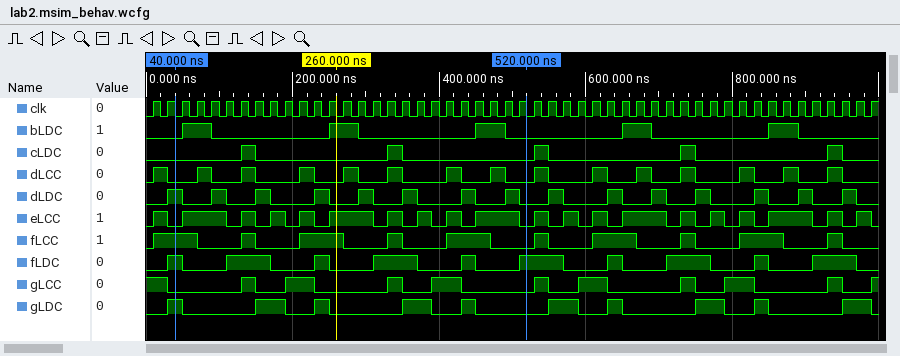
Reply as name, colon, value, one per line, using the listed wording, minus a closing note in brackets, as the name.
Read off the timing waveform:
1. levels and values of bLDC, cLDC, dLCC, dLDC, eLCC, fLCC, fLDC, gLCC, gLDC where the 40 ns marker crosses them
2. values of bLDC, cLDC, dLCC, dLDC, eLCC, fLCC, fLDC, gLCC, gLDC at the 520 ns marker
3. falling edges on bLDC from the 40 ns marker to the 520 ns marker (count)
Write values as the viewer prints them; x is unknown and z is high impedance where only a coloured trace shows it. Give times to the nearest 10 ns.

levels and values of bLDC, cLDC, dLCC, dLDC, eLCC, fLCC, fLDC, gLCC, gLDC where the 40 ns marker crosses them: bLDC=0, cLDC=0, dLCC=0, dLDC=1, eLCC=0, fLCC=1, fLDC=1, gLCC=0, gLDC=1
values of bLDC, cLDC, dLCC, dLDC, eLCC, fLCC, fLDC, gLCC, gLDC at the 520 ns marker: bLDC=0, cLDC=0, dLCC=0, dLDC=0, eLCC=0, fLCC=0, fLDC=1, gLCC=0, gLDC=0
falling edges on bLDC from the 40 ns marker to the 520 ns marker: 3
